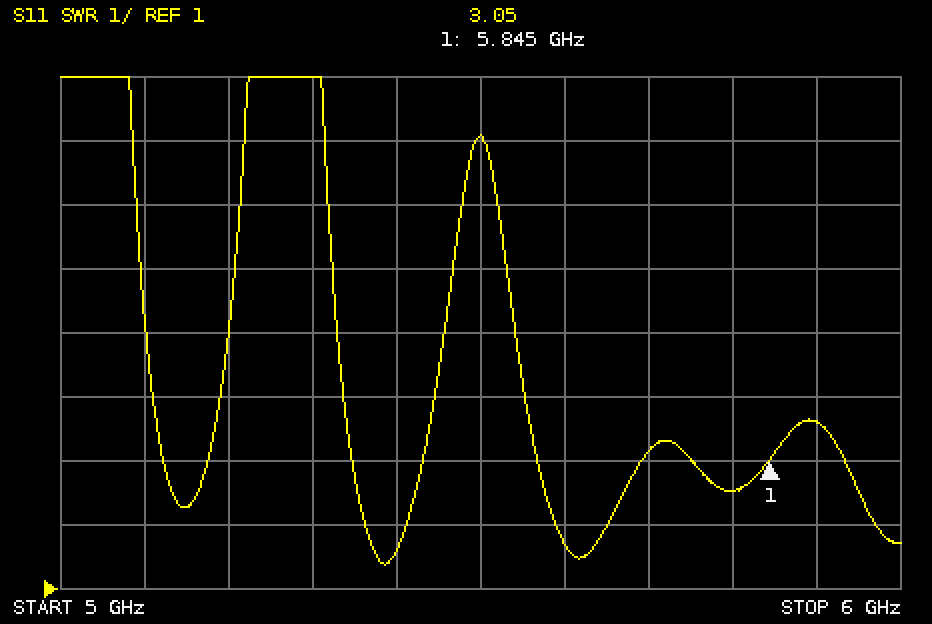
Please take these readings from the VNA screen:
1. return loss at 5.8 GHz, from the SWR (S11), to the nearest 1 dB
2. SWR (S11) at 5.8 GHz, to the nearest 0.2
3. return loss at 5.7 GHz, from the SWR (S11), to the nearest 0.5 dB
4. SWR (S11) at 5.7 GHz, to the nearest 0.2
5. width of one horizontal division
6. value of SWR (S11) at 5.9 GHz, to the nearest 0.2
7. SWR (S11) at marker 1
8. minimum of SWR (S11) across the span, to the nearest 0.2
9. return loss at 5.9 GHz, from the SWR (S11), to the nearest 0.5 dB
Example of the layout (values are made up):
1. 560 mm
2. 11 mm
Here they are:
1. 7 dB
2. 2.6
3. 5.5 dB
4. 3.2
5. 100 MHz
6. 3.6
7. 3.05
8. 1.4
9. 5.0 dB
